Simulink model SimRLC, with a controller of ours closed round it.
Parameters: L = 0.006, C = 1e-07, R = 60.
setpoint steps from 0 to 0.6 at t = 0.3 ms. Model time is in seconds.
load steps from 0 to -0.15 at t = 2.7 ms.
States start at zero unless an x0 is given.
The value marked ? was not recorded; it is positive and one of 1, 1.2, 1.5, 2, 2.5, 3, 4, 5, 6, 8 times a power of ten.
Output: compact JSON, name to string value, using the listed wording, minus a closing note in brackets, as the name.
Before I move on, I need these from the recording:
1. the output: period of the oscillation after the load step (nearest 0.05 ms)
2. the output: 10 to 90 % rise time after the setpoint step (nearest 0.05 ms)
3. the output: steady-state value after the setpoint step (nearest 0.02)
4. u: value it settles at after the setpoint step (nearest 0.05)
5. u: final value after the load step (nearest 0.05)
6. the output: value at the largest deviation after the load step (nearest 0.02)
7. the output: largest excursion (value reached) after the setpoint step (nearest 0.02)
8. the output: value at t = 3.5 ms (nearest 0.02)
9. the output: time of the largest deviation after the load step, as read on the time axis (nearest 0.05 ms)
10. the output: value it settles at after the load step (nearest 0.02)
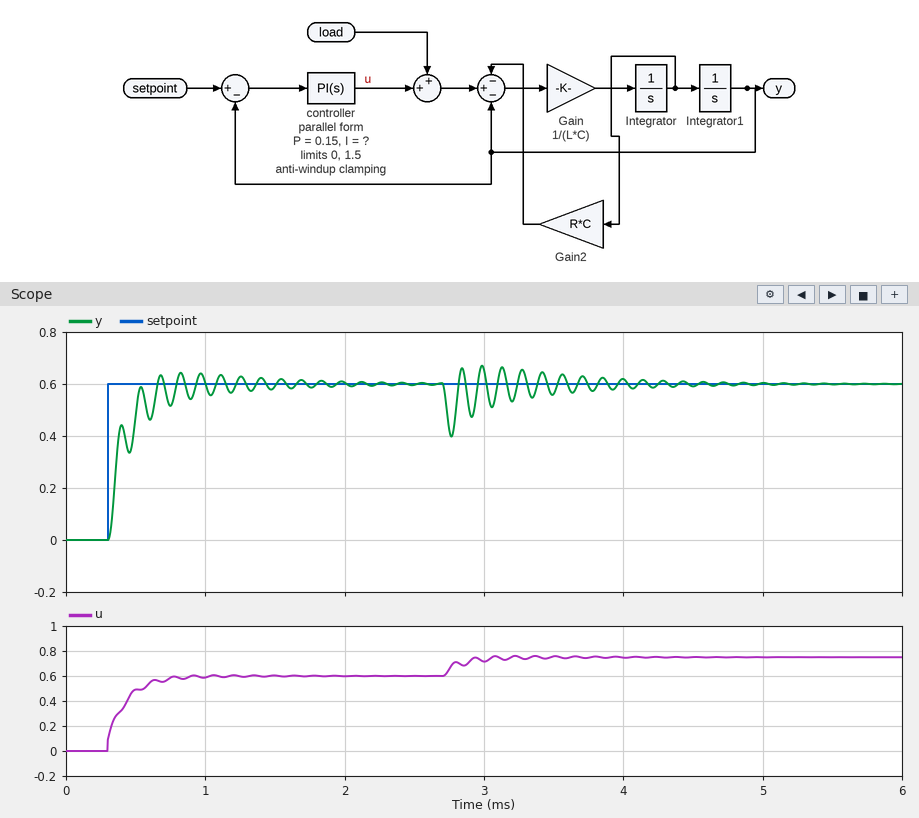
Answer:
{"the output: period of the oscillation after the load step": "0.15 ms", "the output: 10 to 90 % rise time after the setpoint step": "0.20 ms", "the output: steady-state value after the setpoint step": "0.60", "u: value it settles at after the setpoint step": "0.60", "u: final value after the load step": "0.75", "the output: value at the largest deviation after the load step": "0.40", "the output: largest excursion (value reached) after the setpoint step": "0.64", "the output: value at t = 3.5 ms": "0.56", "the output: time of the largest deviation after the load step, as read on the time axis": "2.75 ms", "the output: value it settles at after the load step": "0.60"}
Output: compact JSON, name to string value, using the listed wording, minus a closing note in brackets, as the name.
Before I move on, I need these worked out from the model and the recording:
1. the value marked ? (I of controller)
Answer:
{"the value marked ?": "8000"}
